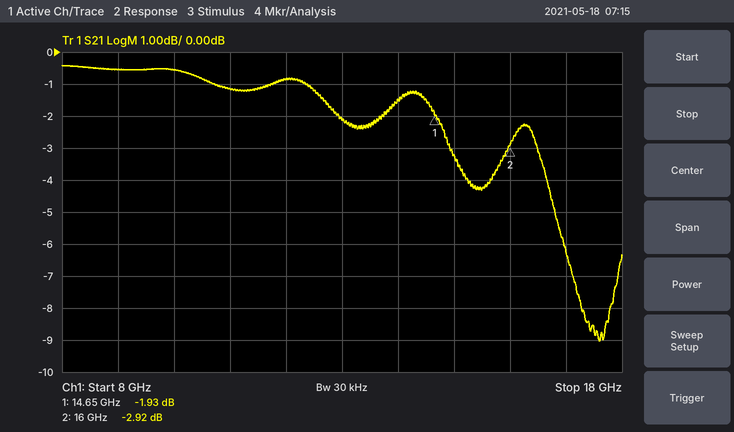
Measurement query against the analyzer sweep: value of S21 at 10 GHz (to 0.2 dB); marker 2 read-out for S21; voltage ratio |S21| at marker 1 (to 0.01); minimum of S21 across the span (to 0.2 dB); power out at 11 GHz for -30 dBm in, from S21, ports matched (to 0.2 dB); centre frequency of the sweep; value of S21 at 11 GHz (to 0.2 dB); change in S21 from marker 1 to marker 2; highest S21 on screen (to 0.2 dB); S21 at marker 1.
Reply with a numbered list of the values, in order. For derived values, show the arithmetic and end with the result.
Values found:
1. -0.6 dB
2. -2.92 dB
3. 10^(-1.93/20) ≈ 0.80
4. -9.0 dB
5. -30 dBm + (-1.2 dB) = -31.2 dBm
6. 13 GHz
7. -1.2 dB
8. -2.92 − (-1.93) = -0.99 dB
9. -0.4 dB
10. -1.93 dB
